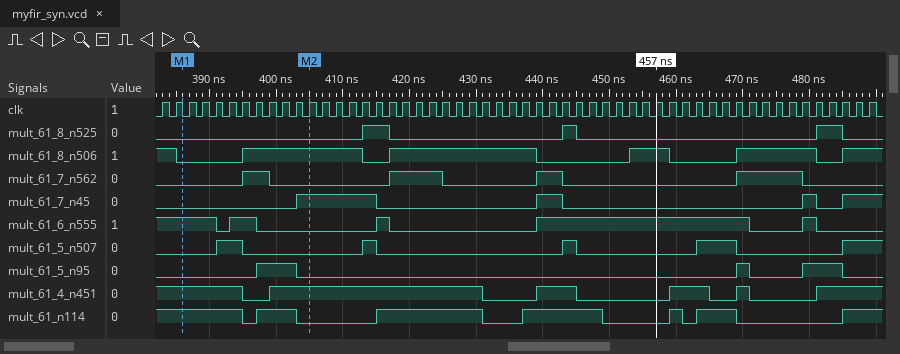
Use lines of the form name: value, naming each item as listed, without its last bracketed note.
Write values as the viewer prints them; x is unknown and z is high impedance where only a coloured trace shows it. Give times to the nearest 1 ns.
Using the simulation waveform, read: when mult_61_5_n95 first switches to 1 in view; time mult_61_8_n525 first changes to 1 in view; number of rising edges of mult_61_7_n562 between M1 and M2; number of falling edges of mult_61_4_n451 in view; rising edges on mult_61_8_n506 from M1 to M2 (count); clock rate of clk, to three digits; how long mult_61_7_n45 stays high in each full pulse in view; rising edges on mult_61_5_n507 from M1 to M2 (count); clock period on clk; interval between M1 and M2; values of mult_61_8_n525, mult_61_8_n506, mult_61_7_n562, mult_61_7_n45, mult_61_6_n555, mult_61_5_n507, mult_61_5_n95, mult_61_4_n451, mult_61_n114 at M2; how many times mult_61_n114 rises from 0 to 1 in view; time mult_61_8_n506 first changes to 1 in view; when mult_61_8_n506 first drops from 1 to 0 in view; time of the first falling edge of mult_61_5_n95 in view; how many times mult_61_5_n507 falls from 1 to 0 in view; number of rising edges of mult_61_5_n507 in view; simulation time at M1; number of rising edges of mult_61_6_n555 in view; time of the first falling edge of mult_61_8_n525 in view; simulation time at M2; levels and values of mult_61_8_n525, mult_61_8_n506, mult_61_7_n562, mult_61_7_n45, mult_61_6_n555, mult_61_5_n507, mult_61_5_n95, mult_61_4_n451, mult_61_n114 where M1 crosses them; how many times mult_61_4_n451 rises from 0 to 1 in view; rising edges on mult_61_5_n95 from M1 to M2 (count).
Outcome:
when mult_61_5_n95 first switches to 1 in view: 397 ns
time mult_61_8_n525 first changes to 1 in view: 413 ns
number of rising edges of mult_61_7_n562 between M1 and M2: 1
number of falling edges of mult_61_4_n451 in view: 5
rising edges on mult_61_8_n506 from M1 to M2: 1
clock rate of clk, to three digits: 500 MHz
how long mult_61_7_n45 stays high in each full pulse in view: 12 ns, 4 ns, 2 ns
rising edges on mult_61_5_n507 from M1 to M2: 1
clock period on clk: 2 ns
interval between M1 and M2: 19 ns
values of mult_61_8_n525, mult_61_8_n506, mult_61_7_n562, mult_61_7_n45, mult_61_6_n555, mult_61_5_n507, mult_61_5_n95, mult_61_4_n451, mult_61_n114 at M2: mult_61_8_n525=0, mult_61_8_n506=1, mult_61_7_n562=0, mult_61_7_n45=1, mult_61_6_n555=0, mult_61_5_n507=0, mult_61_5_n95=0, mult_61_4_n451=1, mult_61_n114=0
how many times mult_61_n114 rises from 0 to 1 in view: 6
time mult_61_8_n506 first changes to 1 in view: 395 ns
when mult_61_8_n506 first drops from 1 to 0 in view: 385 ns
time of the first falling edge of mult_61_5_n95 in view: 403 ns
how many times mult_61_5_n507 falls from 1 to 0 in view: 4
number of rising edges of mult_61_5_n507 in view: 5
simulation time at M1: 386 ns
number of rising edges of mult_61_6_n555 in view: 4
time of the first falling edge of mult_61_8_n525 in view: 417 ns
simulation time at M2: 405 ns
levels and values of mult_61_8_n525, mult_61_8_n506, mult_61_7_n562, mult_61_7_n45, mult_61_6_n555, mult_61_5_n507, mult_61_5_n95, mult_61_4_n451, mult_61_n114 where M1 crosses them: mult_61_8_n525=0, mult_61_8_n506=0, mult_61_7_n562=0, mult_61_7_n45=0, mult_61_6_n555=1, mult_61_5_n507=0, mult_61_5_n95=0, mult_61_4_n451=1, mult_61_n114=1
how many times mult_61_4_n451 rises from 0 to 1 in view: 5
rising edges on mult_61_5_n95 from M1 to M2: 1
